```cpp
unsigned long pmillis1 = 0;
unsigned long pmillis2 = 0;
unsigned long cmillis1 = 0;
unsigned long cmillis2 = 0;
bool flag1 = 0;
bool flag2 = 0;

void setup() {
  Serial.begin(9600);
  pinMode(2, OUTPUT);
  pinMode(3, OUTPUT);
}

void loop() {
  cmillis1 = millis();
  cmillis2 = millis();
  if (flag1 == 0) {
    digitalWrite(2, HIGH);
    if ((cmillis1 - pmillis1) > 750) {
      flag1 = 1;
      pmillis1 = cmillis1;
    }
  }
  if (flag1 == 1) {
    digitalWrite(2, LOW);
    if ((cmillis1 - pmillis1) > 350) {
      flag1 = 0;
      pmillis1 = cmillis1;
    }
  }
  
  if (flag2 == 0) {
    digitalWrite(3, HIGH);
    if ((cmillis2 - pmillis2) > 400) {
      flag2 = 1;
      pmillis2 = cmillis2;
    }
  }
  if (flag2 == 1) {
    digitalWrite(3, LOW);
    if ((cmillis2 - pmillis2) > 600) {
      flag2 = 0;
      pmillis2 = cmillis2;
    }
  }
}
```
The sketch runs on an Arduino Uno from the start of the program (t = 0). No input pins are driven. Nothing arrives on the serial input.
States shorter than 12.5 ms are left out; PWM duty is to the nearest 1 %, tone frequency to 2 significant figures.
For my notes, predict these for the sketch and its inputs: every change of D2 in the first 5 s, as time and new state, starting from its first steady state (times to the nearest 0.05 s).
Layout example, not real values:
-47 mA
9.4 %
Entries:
0 s high; 0.75 s low; 1.1 s high; 1.85 s low; 2.2 s high; 2.95 s low; 3.3 s high; 4.05 s low; 4.4 s high
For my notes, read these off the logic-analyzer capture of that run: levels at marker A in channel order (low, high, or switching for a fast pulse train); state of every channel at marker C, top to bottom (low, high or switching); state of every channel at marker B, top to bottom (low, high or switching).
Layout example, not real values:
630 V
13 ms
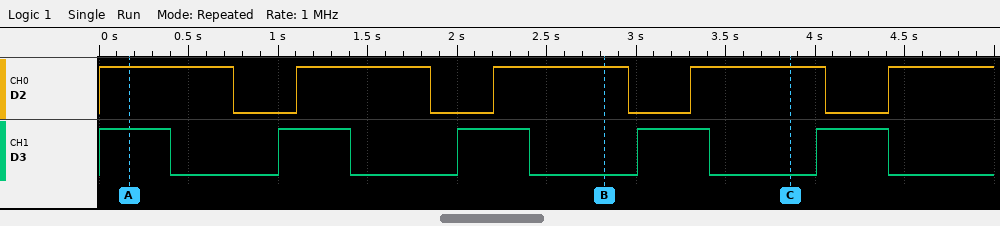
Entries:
D2 high, D3 high
D2 high, D3 low
D2 high, D3 low
